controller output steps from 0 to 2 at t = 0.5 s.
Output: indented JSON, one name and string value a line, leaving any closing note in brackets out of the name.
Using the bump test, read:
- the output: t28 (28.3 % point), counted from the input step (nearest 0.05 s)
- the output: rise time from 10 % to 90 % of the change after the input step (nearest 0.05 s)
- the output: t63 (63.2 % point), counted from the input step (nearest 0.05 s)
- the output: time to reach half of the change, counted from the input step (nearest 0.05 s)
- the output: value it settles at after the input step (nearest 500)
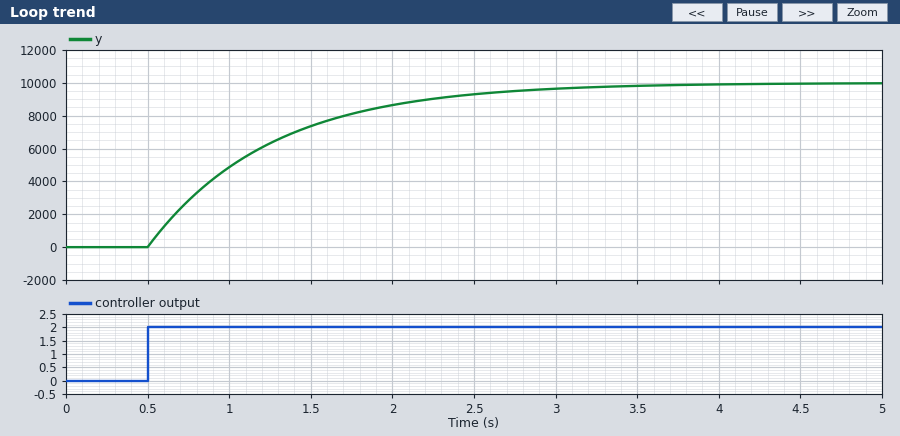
{
  "the output: t28 (28.3 % point), counted from the input step": "0.25 s",
  "the output: rise time from 10 % to 90 % of the change after the input step": "1.65 s",
  "the output: t63 (63.2 % point), counted from the input step": "0.75 s",
  "the output: time to reach half of the change, counted from the input step": "0.50 s",
  "the output: value it settles at after the input step": "10000"
}
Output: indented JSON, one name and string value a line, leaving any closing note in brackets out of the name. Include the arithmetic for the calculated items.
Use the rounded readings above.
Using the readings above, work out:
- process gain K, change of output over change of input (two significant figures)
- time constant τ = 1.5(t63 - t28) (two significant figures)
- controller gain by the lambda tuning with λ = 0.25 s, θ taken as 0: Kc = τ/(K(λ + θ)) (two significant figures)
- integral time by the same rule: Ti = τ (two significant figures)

{
  "process gain K, change of output over change of input": "(10000 - 0) / 2 = 5000",
  "time constant τ = 1.5(t63 - t28)": "1.5 × (0.75 - 0.25) = 0.75 s",
  "controller gain by the lambda tuning with λ = 0.25 s, θ taken as 0: Kc = τ/(K(λ + θ))": "0.75 / (5000 × (0.25 + 0)) = 0.00060",
  "integral time by the same rule: Ti = τ": "0.75 s"
}
